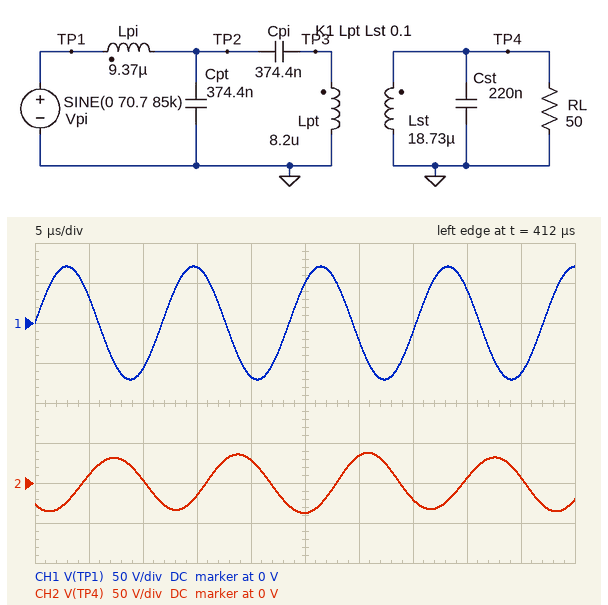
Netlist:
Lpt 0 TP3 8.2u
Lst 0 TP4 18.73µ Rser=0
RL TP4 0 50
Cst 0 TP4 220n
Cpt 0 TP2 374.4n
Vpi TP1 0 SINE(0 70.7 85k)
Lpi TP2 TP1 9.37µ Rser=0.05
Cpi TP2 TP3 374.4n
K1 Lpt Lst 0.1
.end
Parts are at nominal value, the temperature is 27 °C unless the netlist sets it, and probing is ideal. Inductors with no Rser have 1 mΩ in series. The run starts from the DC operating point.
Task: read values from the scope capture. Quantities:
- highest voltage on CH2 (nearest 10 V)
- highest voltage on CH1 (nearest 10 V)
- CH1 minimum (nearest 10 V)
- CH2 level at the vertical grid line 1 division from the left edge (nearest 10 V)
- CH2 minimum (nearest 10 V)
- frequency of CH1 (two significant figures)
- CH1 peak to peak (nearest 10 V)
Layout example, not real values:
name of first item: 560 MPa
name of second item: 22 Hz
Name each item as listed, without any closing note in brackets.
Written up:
highest voltage on CH2: 40 V
highest voltage on CH1: 70 V
CH1 minimum: -70 V
CH2 level at the vertical grid line 1 division from the left edge: 10 V
CH2 minimum: -40 V
frequency of CH1: 85 kHz
CH1 peak to peak: 140 V
